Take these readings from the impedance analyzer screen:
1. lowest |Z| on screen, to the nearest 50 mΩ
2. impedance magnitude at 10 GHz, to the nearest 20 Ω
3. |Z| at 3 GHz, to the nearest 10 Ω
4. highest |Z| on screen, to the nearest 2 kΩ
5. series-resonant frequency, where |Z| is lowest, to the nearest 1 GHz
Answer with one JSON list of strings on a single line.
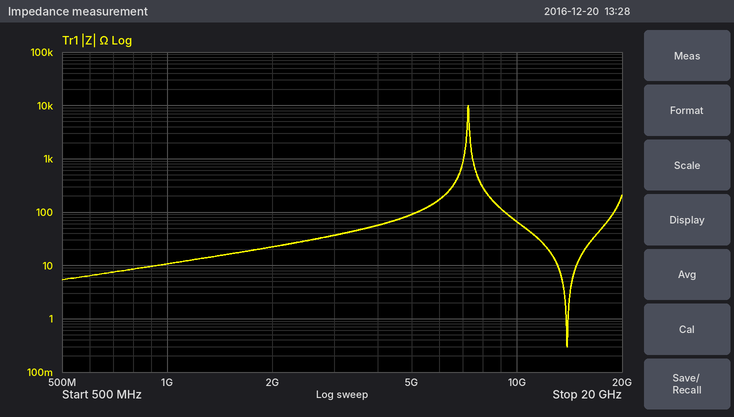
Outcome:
["300 mΩ", "60 Ω", "40 Ω", "10 kΩ", "14 GHz"]
